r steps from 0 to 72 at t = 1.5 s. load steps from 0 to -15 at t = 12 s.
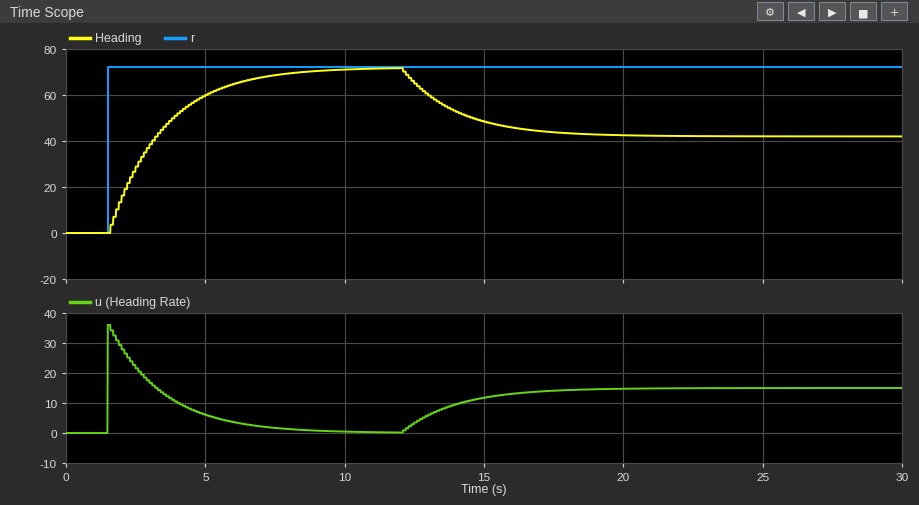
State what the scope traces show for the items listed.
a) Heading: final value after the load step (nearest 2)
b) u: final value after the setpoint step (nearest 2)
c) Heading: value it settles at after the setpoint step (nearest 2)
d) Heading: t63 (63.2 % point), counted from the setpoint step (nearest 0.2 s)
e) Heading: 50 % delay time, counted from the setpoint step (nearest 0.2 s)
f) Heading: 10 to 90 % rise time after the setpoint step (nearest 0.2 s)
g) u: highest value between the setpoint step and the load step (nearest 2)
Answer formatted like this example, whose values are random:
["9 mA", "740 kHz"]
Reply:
["42", "0", "72", "2.0 s", "1.4 s", "4.2 s", "36"]
